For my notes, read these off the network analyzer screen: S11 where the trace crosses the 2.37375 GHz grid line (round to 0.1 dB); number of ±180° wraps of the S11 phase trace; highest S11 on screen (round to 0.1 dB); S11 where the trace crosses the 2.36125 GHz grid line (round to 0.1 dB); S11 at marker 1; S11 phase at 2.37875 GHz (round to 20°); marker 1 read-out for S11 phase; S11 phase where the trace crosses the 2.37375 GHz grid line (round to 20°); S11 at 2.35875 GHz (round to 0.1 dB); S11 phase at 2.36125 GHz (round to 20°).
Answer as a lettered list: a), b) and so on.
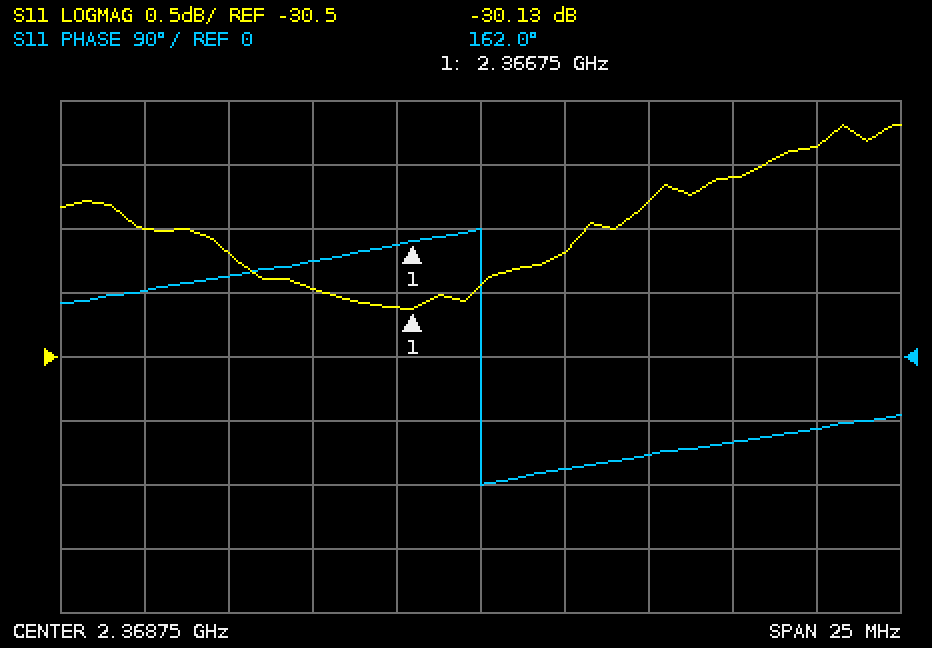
a) -29.3 dB
b) 1
c) -28.7 dB
d) -29.7 dB
e) -30.13 dB
f) -100°
g) 162.0°
h) -140°
i) -29.5 dB
j) 120°
